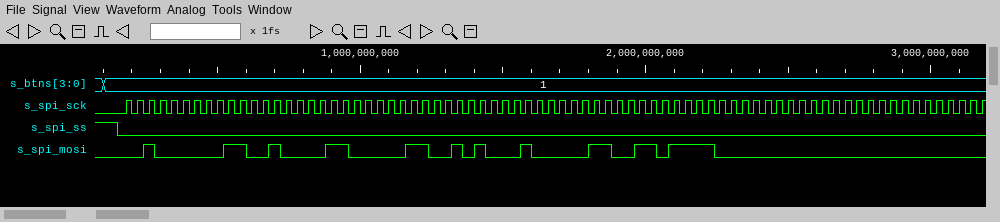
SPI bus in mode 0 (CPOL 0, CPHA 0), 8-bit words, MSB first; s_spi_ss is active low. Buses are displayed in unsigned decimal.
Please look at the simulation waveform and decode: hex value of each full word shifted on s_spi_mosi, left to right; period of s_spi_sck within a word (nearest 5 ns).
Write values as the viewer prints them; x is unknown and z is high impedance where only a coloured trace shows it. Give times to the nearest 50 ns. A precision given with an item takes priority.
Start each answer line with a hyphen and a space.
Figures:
- 20, 64, 30, 65, 10, 66, F0, 00, 00
- 40 ns
